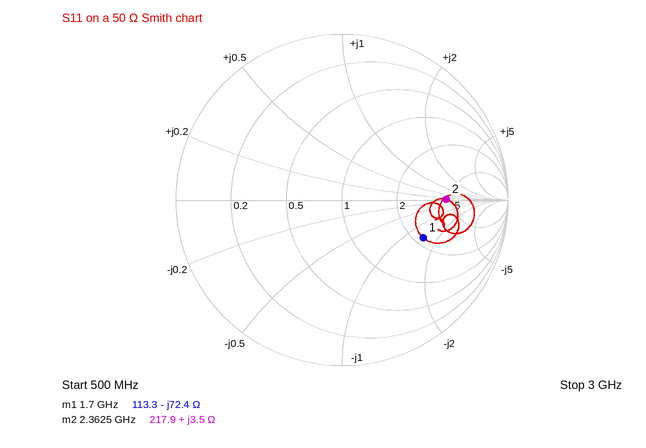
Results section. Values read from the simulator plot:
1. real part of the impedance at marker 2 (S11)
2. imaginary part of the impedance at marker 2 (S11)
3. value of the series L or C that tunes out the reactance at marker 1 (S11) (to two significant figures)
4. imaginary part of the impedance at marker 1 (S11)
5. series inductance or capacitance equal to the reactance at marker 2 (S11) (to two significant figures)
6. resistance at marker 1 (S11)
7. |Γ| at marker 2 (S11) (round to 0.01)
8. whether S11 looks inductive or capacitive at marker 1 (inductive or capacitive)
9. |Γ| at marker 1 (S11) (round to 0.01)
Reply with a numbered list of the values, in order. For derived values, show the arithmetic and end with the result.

1. 217.9 Ω
2. +3.5 Ω
3. L = 72.4 Ω/(2π × 1.7 GHz) ≈ 6.8 nH
4. -72.4 Ω
5. L = 3.5 Ω/(2π × 2.3625 GHz) ≈ 236 pH, so 240 pH to two significant figures
6. 113.3 Ω
7. 0.63
8. capacitive
9. 0.54
